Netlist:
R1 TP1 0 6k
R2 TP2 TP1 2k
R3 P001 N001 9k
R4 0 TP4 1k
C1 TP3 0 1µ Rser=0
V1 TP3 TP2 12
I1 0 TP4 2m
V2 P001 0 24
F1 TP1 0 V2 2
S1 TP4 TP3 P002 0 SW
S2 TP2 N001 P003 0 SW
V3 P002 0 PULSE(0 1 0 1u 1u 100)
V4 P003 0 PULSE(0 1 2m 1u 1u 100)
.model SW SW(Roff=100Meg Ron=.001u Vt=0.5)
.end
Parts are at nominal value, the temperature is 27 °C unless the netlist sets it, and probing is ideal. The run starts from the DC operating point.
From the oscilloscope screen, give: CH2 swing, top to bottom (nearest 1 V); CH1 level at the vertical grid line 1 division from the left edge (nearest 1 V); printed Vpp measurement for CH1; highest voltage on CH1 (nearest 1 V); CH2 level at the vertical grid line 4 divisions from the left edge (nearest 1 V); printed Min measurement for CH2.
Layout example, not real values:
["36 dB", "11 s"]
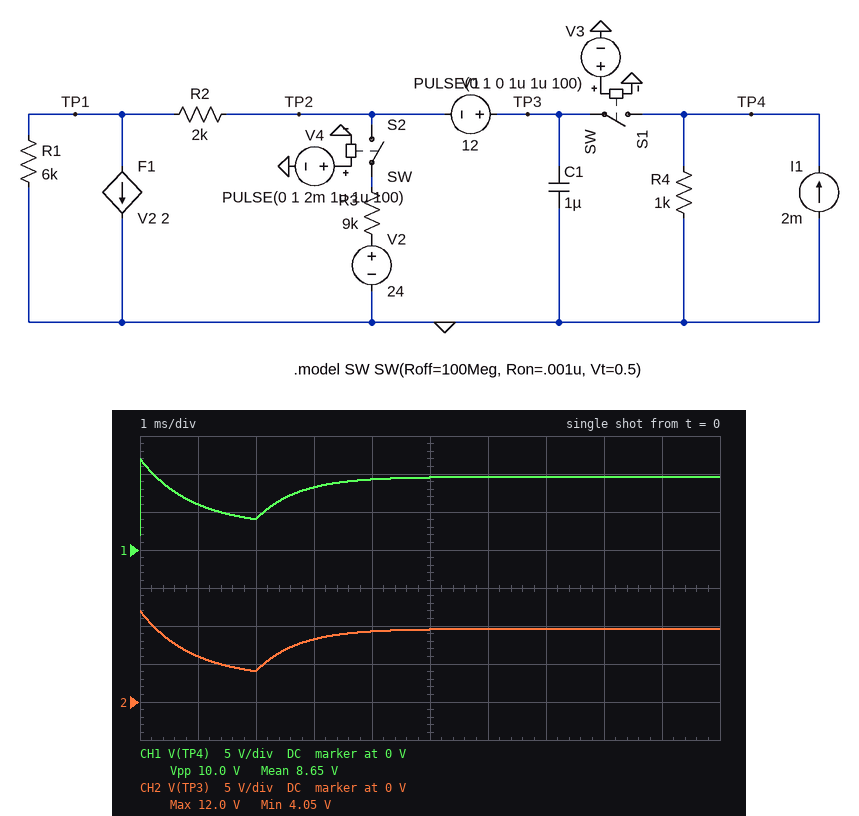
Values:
["8 V", "6 V", "10.0 V", "12 V", "9 V", "4.05 V"]
